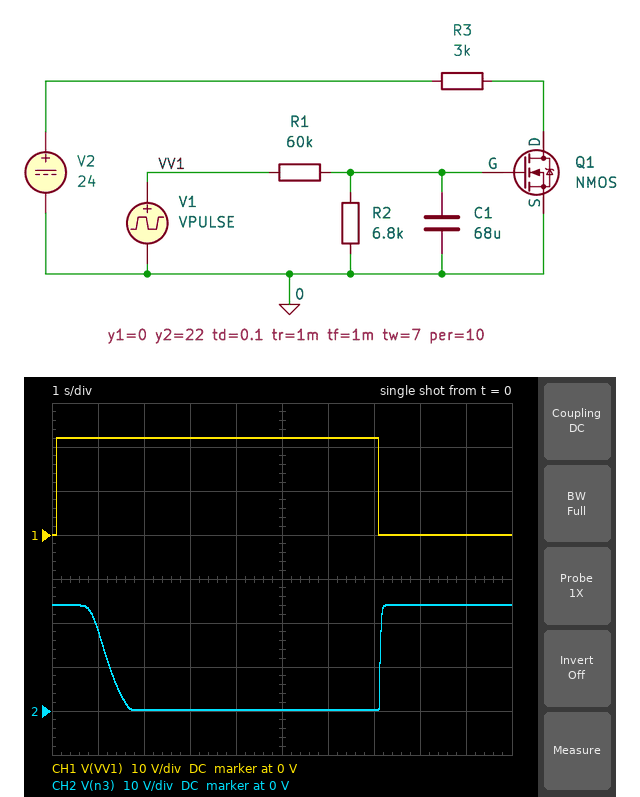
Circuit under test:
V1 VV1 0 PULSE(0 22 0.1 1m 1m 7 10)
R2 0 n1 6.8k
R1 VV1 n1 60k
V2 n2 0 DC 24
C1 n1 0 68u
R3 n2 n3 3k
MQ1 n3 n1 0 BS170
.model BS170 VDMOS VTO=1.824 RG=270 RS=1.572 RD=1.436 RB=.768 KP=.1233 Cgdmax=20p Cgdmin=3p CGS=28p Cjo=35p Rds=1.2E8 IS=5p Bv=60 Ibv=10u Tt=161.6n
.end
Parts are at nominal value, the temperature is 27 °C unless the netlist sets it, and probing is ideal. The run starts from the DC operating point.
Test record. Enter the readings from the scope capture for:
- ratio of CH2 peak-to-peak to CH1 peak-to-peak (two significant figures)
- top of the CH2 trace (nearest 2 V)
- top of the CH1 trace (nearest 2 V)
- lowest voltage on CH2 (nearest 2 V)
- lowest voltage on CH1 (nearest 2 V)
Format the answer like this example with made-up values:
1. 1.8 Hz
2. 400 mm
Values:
1. 1.1
2. 24 V
3. 22 V
4. 0 V
5. 0 V
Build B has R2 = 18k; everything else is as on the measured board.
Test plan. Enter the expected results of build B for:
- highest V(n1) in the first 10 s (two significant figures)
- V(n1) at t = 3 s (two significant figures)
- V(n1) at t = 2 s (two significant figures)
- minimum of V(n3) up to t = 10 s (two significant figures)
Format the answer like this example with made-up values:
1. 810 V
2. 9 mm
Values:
1. 5.1 V
2. 4.8 V
3. 4.4 V
4. 44 mV
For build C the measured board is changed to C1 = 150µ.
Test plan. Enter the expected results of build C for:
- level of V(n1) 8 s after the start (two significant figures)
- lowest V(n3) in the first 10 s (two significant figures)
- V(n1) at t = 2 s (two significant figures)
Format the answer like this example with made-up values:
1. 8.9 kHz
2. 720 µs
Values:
1. 840 mV
2. 240 mV
3. 2.0 V
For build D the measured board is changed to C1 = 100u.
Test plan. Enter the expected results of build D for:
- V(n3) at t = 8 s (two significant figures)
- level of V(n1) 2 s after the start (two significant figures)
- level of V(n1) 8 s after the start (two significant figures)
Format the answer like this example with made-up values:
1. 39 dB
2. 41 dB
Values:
1. 24 V
2. 2.1 V
3. 510 mV
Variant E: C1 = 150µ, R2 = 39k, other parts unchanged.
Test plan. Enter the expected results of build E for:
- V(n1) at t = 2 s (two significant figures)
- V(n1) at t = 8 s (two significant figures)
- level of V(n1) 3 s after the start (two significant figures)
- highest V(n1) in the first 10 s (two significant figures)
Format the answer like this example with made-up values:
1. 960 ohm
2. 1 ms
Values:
1. 3.6 V
2. 5.8 V
3. 4.8 V
4. 7.5 V
